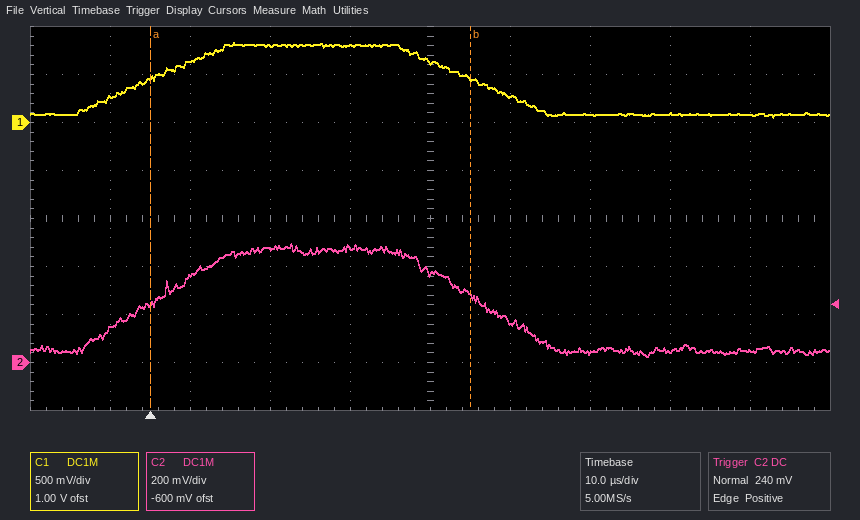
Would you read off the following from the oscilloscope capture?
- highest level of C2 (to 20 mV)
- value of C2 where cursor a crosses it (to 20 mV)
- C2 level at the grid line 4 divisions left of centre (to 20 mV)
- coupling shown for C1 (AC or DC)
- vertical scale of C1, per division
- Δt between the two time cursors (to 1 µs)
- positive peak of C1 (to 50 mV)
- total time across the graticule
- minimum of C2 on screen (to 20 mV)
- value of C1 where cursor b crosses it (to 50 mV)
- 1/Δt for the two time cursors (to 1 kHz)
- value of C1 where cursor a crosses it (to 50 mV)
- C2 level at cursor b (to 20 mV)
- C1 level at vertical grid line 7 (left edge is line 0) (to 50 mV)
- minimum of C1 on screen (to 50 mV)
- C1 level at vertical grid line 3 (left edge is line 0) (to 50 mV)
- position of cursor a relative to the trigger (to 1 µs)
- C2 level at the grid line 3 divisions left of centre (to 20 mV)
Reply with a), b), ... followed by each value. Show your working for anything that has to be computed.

a) 500 mV
b) 240 mV
c) 140 mV
d) DC
e) 500 mV
f) 40 µs
g) 850 mV
h) 100 µs
i) 20 mV
j) 450 mV
k) 1 / 40 µs ≈ 25 kHz
l) 450 mV
m) 280 mV
n) 100 mV
o) 50 mV
p) 800 mV
q) 0 µs
r) 360 mV
